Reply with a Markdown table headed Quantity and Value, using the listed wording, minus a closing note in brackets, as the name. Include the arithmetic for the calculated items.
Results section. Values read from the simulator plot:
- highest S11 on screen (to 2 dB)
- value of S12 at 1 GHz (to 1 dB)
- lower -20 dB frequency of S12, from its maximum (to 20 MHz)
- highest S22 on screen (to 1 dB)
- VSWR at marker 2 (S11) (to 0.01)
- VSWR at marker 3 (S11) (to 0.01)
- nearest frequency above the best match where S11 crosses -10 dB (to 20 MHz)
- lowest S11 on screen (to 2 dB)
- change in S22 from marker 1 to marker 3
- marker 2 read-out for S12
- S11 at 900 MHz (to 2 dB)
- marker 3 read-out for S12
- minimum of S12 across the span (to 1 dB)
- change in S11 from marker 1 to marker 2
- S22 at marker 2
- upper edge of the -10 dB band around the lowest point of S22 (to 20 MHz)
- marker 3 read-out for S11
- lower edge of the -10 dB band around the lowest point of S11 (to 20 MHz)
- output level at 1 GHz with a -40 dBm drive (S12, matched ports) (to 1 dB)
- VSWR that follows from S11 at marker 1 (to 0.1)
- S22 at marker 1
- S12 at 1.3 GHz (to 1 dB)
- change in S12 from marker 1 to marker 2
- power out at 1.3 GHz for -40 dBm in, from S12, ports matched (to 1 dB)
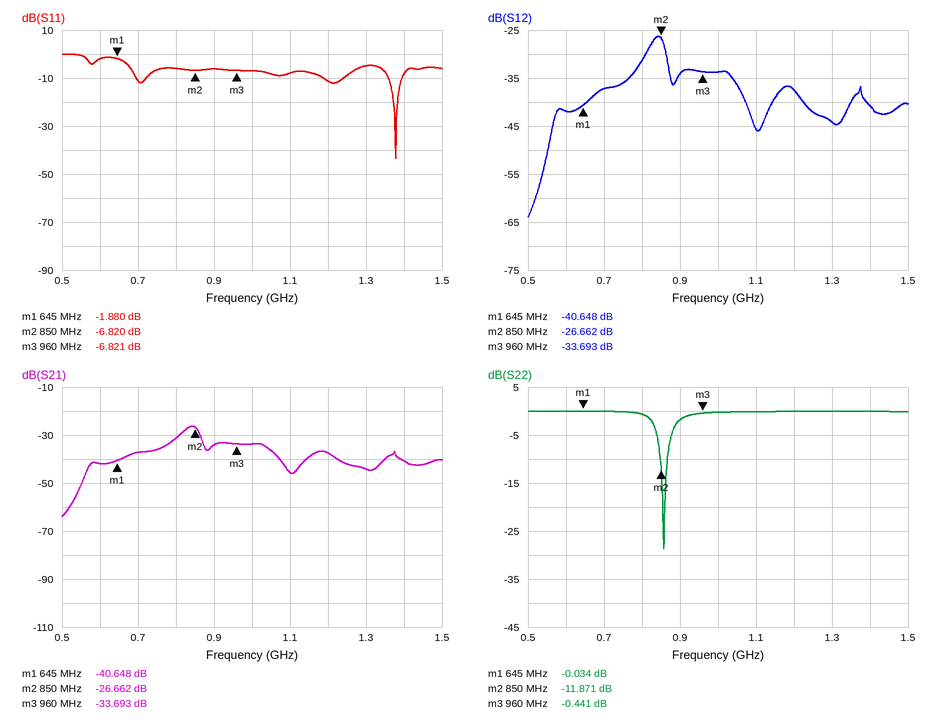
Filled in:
| Quantity | Value |
|---|---|
| highest S11 on screen | 0 dB |
| value of S12 at 1 GHz | -34 dB |
| lower -20 dB frequency of S12, from its maximum | 560 MHz |
| highest S22 on screen | 0 dB |
| VSWR at marker 2 (S11) | (1 + 0.4560)/(1 − 0.4560) ≈ 2.68 |
| VSWR at marker 3 (S11) | (1 + 0.4560)/(1 − 0.4560) ≈ 2.68 |
| nearest frequency above the best match where S11 crosses -10 dB | 1.40 GHz |
| lowest S11 on screen | -44 dB |
| change in S22 from marker 1 to marker 3 | -0.441 − (-0.034) = -0.407 dB |
| marker 2 read-out for S12 | -26.662 dB |
| S11 at 900 MHz | -6 dB |
| marker 3 read-out for S12 | -33.693 dB |
| minimum of S12 across the span | -64 dB |
| change in S11 from marker 1 to marker 2 | -6.82 − (-1.88) = -4.940 dB |
| S22 at marker 2 | -11.871 dB |
| upper edge of the -10 dB band around the lowest point of S22 | 860 MHz |
| marker 3 read-out for S11 | -6.821 dB |
| lower edge of the -10 dB band around the lowest point of S11 | 1.36 GHz |
| output level at 1 GHz with a -40 dBm drive (S12, matched ports) | -40 dBm + (-34 dB) = -74 dBm |
| VSWR that follows from S11 at marker 1 | (1 + 0.8054)/(1 − 0.8054) ≈ 9.3 |
| S22 at marker 1 | -0.034 dB |
| S12 at 1.3 GHz | -44 dB |
| change in S12 from marker 1 to marker 2 | -26.662 − (-40.648) = 13.986 dB |
| power out at 1.3 GHz for -40 dBm in, from S12, ports matched | -40 dBm + (-44 dB) = -84 dBm |
